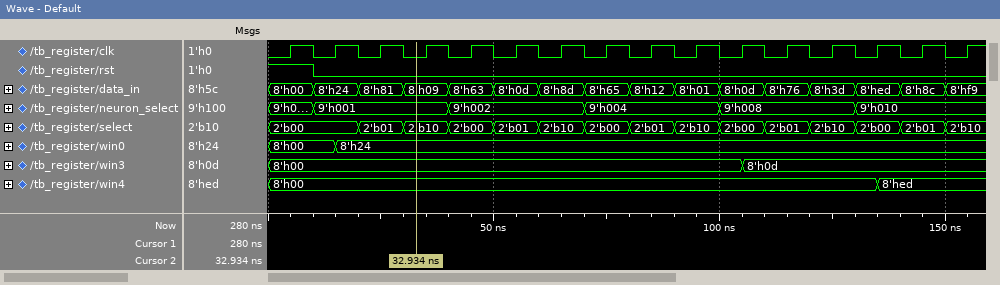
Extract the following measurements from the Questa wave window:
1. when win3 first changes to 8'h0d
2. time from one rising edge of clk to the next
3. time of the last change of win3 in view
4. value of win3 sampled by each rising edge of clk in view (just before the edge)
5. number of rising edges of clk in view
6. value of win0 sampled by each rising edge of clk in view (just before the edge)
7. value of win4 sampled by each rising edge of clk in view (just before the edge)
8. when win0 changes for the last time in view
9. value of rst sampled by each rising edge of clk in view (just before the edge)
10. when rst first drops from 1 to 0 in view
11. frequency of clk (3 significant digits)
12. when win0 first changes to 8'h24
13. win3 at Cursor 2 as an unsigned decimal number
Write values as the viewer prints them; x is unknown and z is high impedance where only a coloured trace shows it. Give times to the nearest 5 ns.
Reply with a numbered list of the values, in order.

1. 105 ns
2. 10 ns
3. 105 ns
4. 8'h00, 8'h00, 8'h00, 8'h00, 8'h00, 8'h00, 8'h00, 8'h00, 8'h00, 8'h00, 8'h00, 8'h0d, 8'h0d, 8'h0d, 8'h0d, 8'h0d
5. 16
6. 8'h00, 8'h00, 8'h24, 8'h24, 8'h24, 8'h24, 8'h24, 8'h24, 8'h24, 8'h24, 8'h24, 8'h24, 8'h24, 8'h24, 8'h24, 8'h24
7. 8'h00, 8'h00, 8'h00, 8'h00, 8'h00, 8'h00, 8'h00, 8'h00, 8'h00, 8'h00, 8'h00, 8'h00, 8'h00, 8'h00, 8'hed, 8'hed
8. 15 ns
9. 1 0 0 0 0 0 0 0 0 0 0 0 0 0 0 0
10. 10 ns
11. 100 MHz
12. 15 ns
13. 0
